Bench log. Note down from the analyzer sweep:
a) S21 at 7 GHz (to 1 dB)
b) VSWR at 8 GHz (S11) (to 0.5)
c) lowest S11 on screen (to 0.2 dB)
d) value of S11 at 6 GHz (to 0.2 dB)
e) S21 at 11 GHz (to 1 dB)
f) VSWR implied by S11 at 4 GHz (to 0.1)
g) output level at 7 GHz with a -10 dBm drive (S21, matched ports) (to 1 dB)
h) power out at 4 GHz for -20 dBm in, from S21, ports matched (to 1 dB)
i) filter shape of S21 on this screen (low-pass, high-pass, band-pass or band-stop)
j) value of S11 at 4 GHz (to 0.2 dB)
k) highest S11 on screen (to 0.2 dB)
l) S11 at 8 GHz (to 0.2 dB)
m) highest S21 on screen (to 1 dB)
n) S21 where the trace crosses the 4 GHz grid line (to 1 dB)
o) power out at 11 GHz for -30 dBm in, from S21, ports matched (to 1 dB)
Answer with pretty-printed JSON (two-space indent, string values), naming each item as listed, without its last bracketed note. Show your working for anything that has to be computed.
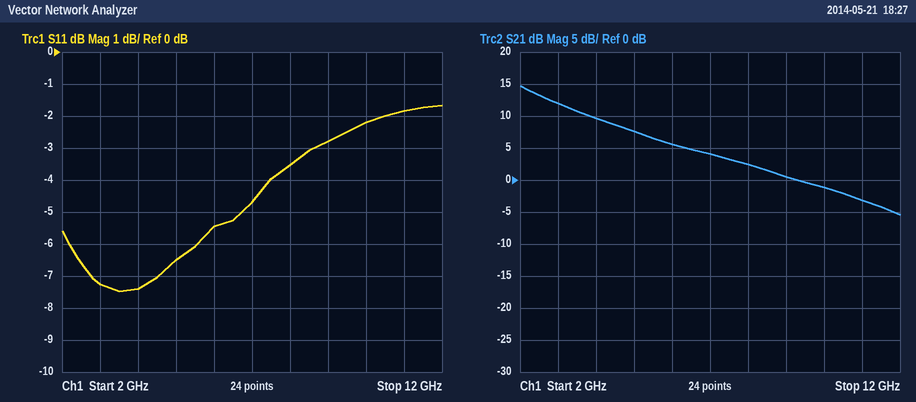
{
  "S21 at 7 GHz": "4 dB",
  "VSWR at 8 GHz (S11)": "|Γ| = 10^(-3.6/20) = 0.6607; VSWR = (1 + 0.6607)/(1 − 0.6607) ≈ 4.89, so 5.0 to the nearest 0.5",
  "lowest S11 on screen": "-7.4 dB",
  "value of S11 at 6 GHz": "-5.4 dB",
  "S21 at 11 GHz": "-3 dB",
  "VSWR implied by S11 at 4 GHz": "|Γ| = 10^(-7.4/20) = 0.4266; VSWR = (1 + 0.4266)/(1 − 0.4266) ≈ 2.5",
  "output level at 7 GHz with a -10 dBm drive (S21, matched ports)": "-10 dBm + (4 dB) = -6 dBm",
  "power out at 4 GHz for -20 dBm in, from S21, ports matched": "-20 dBm + (10 dB) = -10 dBm",
  "filter shape of S21 on this screen": "low-pass",
  "value of S11 at 4 GHz": "-7.4 dB",
  "highest S11 on screen": "-1.6 dB",
  "S11 at 8 GHz": "-3.6 dB",
  "highest S21 on screen": "15 dB",
  "S21 where the trace crosses the 4 GHz grid line": "10 dB",
  "power out at 11 GHz for -30 dBm in, from S21, ports matched": "-30 dBm + (-3 dB) = -33 dBm"
}
